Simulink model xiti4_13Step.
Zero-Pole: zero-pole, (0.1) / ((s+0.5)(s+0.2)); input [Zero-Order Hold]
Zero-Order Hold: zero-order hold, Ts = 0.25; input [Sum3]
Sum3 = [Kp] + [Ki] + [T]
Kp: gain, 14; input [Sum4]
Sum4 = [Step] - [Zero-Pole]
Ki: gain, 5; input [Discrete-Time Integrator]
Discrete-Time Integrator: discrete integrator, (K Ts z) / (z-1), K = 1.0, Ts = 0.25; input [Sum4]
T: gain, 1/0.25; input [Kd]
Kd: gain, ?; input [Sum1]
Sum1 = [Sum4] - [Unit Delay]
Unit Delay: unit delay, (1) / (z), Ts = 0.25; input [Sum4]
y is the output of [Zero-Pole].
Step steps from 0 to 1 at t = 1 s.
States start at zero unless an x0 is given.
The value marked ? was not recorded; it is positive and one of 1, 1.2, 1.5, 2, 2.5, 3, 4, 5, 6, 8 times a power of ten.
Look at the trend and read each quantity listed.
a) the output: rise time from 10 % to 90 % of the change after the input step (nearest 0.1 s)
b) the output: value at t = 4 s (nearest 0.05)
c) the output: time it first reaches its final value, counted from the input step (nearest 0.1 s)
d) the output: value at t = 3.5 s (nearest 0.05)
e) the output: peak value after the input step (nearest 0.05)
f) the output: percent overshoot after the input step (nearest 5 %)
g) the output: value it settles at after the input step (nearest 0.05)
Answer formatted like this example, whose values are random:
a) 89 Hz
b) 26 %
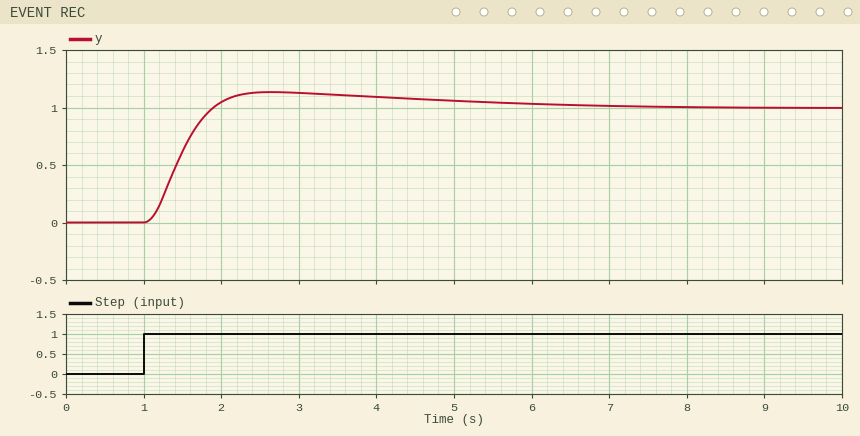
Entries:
a) 0.6 s
b) 1.10
c) 0.9 s
d) 1.10
e) 1.15
f) 15 %
g) 1.00
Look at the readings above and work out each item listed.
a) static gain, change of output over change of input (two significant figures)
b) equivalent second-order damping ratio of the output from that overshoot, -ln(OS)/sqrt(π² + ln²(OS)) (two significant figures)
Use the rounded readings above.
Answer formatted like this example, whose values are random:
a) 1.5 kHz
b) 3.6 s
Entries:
a) 1.0
b) 0.52
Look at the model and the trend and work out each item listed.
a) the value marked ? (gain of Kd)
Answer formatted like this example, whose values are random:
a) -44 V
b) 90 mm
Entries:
a) 15
